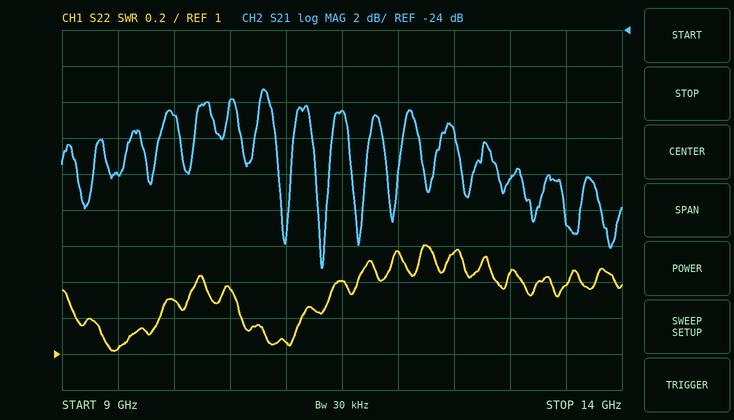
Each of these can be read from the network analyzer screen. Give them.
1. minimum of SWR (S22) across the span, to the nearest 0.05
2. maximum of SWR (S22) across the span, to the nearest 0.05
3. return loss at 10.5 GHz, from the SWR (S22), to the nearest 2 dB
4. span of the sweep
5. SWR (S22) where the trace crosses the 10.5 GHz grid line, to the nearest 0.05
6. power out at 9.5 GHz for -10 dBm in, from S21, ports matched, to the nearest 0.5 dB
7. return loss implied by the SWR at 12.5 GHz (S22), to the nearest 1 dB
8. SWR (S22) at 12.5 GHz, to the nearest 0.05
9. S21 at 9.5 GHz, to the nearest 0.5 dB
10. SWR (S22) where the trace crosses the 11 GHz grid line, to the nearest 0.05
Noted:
1.00
1.60
16 dB
5 GHz
1.35
-42.0 dBm
13 dB
1.55
-32.0 dB
1.05
